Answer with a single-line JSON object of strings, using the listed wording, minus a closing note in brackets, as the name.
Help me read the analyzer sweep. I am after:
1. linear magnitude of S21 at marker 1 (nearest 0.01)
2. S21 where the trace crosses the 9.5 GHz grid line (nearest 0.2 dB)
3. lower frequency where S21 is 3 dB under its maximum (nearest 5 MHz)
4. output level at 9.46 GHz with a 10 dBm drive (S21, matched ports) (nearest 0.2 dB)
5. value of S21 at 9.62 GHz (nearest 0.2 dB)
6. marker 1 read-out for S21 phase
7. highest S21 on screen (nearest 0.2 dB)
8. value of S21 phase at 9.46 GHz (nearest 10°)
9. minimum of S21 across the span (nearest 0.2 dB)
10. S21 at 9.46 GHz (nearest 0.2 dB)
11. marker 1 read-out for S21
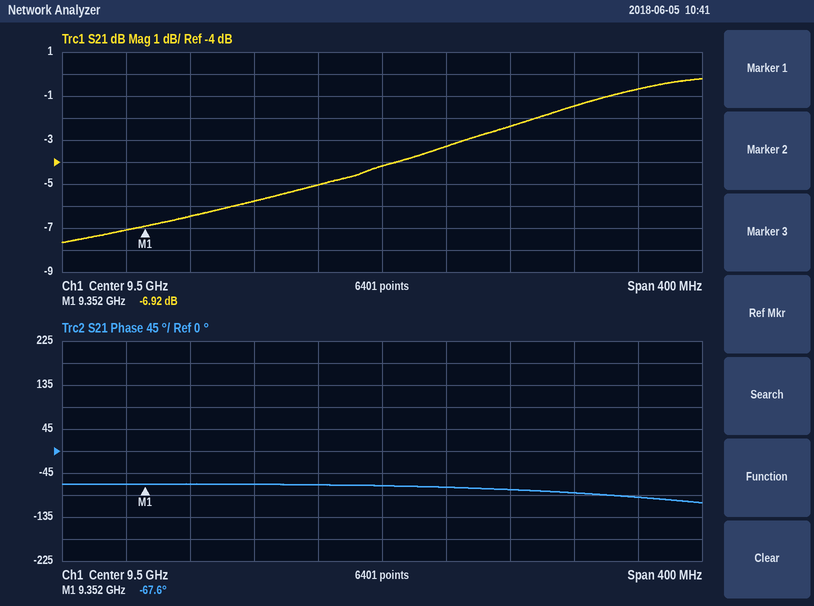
{"linear magnitude of S21 at marker 1": "0.45", "S21 where the trace crosses the 9.5 GHz grid line": "-4.2 dB", "lower frequency where S21 is 3 dB under its maximum": "9.545 GHz", "output level at 9.46 GHz with a 10 dBm drive (S21, matched ports)": "5.0 dBm", "value of S21 at 9.62 GHz": "-1.4 dB", "marker 1 read-out for S21 phase": "-67.6°", "highest S21 on screen": "-0.2 dB", "value of S21 phase at 9.46 GHz": "-70°", "minimum of S21 across the span": "-7.6 dB", "S21 at 9.46 GHz": "-5.0 dB", "marker 1 read-out for S21": "-6.92 dB"}
